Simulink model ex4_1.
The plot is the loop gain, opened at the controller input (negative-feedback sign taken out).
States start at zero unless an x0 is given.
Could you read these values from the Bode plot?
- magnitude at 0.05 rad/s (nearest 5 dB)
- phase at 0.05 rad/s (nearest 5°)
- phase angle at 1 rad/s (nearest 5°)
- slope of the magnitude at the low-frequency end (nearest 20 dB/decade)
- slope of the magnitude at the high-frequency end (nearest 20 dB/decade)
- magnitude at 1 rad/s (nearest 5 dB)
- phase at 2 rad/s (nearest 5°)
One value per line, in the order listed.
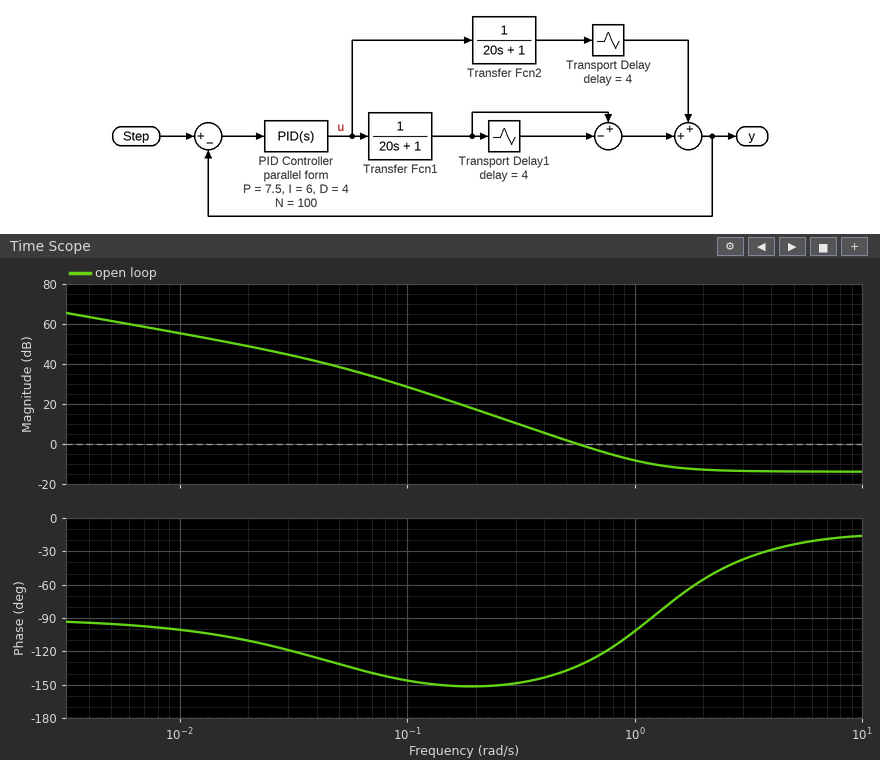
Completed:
40 dB
-130°
-100°
-20 dB/decade
0 dB/decade
-10 dB
-55°
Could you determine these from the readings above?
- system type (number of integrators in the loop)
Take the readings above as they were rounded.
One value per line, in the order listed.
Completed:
1
